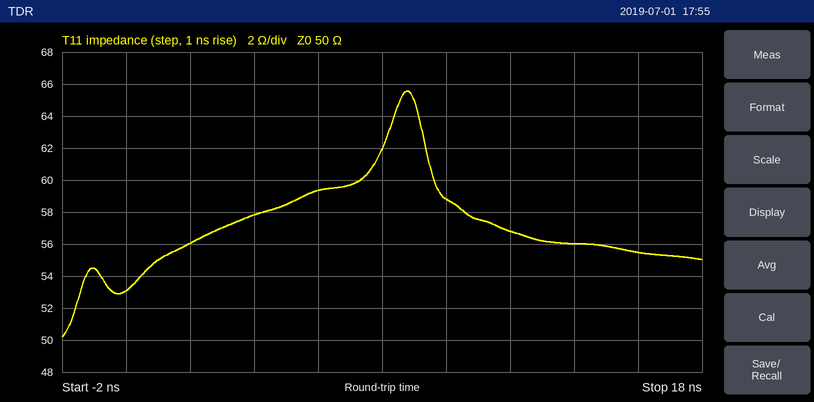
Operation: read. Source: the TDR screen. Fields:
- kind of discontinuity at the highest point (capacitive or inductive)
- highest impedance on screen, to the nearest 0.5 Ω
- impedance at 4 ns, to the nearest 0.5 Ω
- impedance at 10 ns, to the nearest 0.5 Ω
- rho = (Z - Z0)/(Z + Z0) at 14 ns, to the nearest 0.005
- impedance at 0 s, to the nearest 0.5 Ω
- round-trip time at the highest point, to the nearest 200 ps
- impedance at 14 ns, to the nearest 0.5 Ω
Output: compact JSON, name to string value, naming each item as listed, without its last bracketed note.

{"kind of discontinuity at the highest point": "inductive", "highest impedance on screen, to the nearest 0.5 Ω": "65.5 Ω", "impedance at 4 ns, to the nearest 0.5 Ω": "58.0 Ω", "impedance at 10 ns, to the nearest 0.5 Ω": "59.0 Ω", "rho = (Z - Z0)/(Z + Z0) at 14 ns, to the nearest 0.005": "+0.055", "impedance at 0 s, to the nearest 0.5 Ω": "53.0 Ω", "round-trip time at the highest point, to the nearest 200 ps": "8.8 ns", "impedance at 14 ns, to the nearest 0.5 Ω": "56.0 Ω"}
